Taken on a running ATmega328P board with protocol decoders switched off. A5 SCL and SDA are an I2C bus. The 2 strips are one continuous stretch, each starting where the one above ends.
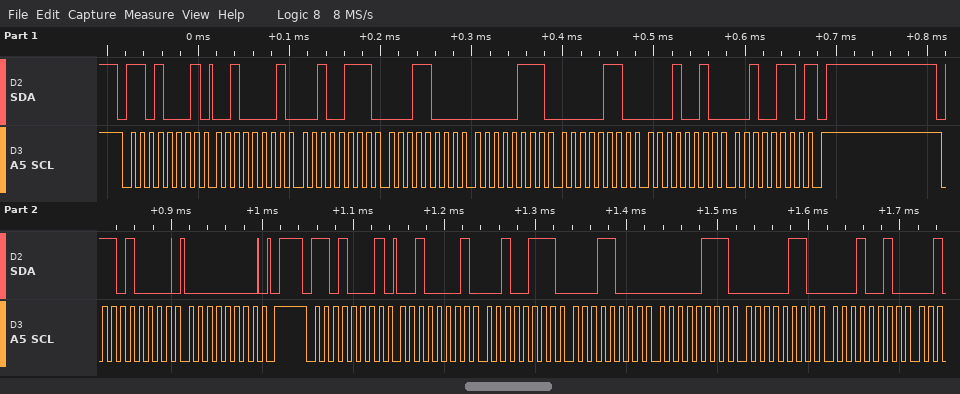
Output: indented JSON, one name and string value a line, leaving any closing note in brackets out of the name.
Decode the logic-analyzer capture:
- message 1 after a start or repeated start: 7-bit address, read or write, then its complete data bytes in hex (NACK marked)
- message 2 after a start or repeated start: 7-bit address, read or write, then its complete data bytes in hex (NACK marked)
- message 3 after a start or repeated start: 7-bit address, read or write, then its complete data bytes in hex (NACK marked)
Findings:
{
  "message 1 after a start or repeated start: 7-bit address, read or write, then its complete data bytes in hex": "0x68 read: 21 27 18 07 06 12 26 NACK",
  "message 2 after a start or repeated start: 7-bit address, read or write, then its complete data bytes in hex": "0x68 write: 00",
  "message 3 after a start or repeated start: 7-bit address, read or write, then its complete data bytes in hex": "0x68 read: 21 27 18 07 06 12"
}
